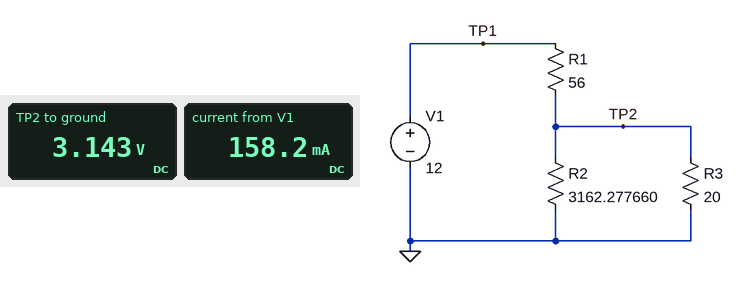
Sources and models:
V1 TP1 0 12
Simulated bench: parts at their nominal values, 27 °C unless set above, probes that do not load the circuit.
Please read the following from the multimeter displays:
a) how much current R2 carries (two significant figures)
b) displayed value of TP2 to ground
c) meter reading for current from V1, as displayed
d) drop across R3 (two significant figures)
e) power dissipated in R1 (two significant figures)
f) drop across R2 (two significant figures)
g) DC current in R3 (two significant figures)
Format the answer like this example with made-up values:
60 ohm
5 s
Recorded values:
990 µA
3.143 V
158.2 mA
3.1 V
1.4 W
3.1 V
160 mA
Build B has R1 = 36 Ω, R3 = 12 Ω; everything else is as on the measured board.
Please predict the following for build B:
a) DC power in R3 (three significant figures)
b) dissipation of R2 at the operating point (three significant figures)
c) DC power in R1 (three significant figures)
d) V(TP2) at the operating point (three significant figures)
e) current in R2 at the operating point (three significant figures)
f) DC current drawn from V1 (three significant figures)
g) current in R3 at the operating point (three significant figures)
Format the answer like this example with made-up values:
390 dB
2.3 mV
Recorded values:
746 mW
2.83 mW
2.25 W
2.99 V
946 µA
250 mA
249 mA
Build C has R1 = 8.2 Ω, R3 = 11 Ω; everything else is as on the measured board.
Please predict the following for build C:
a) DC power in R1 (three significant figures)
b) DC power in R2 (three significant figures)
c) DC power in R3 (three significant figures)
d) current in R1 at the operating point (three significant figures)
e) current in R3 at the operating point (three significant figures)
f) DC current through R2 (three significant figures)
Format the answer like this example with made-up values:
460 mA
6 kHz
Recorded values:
3.22 W
14.9 mW
4.28 W
626 mA
624 mA
2.17 mA
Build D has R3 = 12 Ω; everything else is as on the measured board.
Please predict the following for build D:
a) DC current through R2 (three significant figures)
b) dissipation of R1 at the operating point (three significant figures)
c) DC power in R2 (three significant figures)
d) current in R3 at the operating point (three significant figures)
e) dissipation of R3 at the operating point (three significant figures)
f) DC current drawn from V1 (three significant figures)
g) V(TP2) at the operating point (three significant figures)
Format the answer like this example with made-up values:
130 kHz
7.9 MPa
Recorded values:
668 µA
1.75 W
1.41 mW
176 mA
371 mW
177 mA
2.11 V
